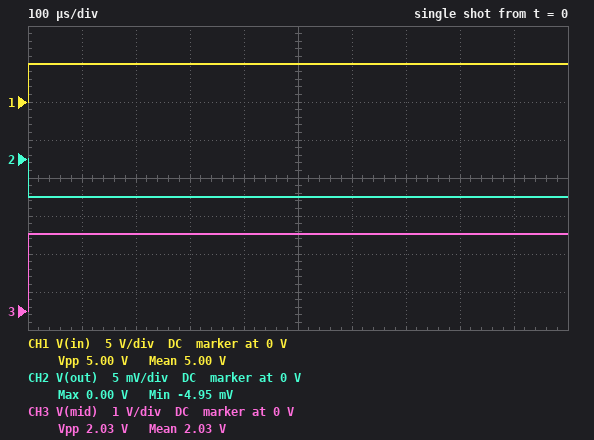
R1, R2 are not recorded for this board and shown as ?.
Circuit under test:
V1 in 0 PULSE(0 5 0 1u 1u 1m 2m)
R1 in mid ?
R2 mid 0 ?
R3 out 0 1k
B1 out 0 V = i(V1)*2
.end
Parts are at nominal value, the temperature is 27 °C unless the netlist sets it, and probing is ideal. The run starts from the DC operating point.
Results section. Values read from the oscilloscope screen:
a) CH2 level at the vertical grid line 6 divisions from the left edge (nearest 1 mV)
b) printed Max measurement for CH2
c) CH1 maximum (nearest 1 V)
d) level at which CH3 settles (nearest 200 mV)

-5 mV
0.00 V
5 V
2.0 V
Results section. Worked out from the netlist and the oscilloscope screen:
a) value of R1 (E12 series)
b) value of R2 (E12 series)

1.2 kΩ
820 Ω
